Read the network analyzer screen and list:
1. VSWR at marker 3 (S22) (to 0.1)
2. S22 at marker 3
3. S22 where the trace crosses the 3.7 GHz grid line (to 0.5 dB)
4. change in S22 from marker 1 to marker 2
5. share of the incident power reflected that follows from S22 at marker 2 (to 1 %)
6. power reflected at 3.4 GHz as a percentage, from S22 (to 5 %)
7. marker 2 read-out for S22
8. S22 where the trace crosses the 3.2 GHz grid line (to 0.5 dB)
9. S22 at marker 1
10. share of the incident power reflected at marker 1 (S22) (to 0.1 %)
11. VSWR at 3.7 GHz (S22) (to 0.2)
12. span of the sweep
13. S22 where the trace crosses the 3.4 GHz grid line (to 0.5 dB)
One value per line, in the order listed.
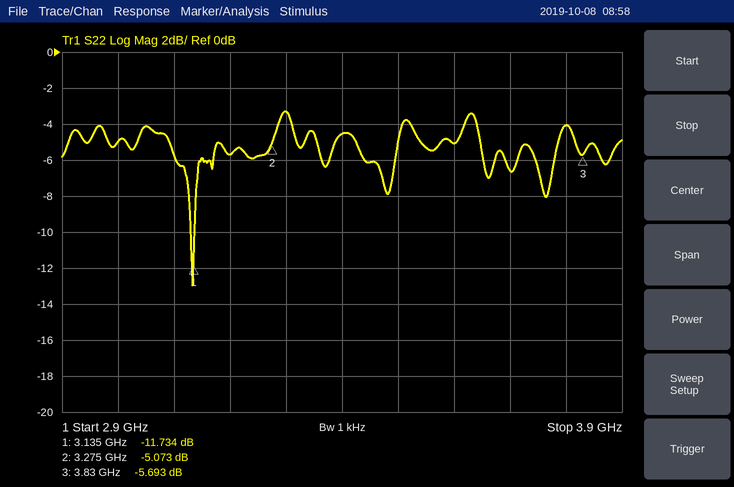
3.2
-5.693 dB
-6.5 dB
6.661 dB
31 %
35 %
-5.073 dB
-5.5 dB
-11.734 dB
6.7 %
2.8
1 GHz
-4.5 dB
